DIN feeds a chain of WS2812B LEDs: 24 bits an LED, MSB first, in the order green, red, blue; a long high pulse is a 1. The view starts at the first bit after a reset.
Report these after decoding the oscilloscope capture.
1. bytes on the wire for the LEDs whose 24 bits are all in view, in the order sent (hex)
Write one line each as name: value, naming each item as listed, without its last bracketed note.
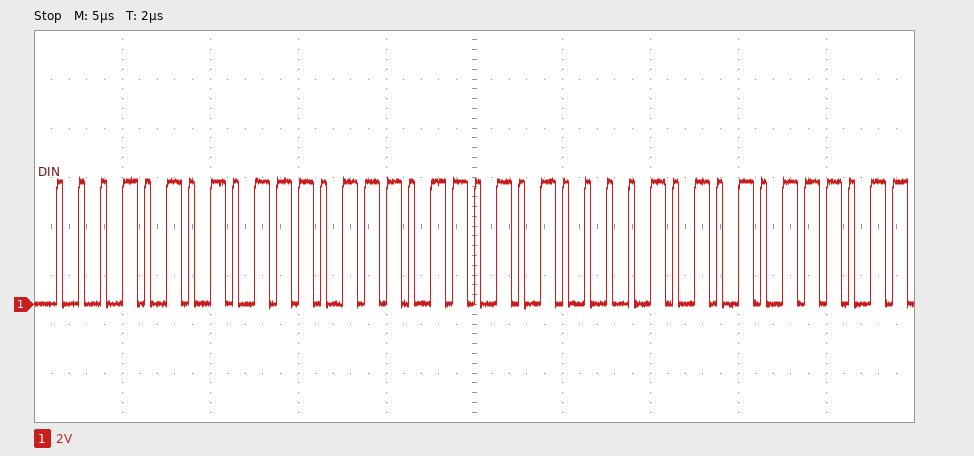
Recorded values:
bytes on the wire for the LEDs whose 24 bits are all in view, in the order sent: 15 77 6A
